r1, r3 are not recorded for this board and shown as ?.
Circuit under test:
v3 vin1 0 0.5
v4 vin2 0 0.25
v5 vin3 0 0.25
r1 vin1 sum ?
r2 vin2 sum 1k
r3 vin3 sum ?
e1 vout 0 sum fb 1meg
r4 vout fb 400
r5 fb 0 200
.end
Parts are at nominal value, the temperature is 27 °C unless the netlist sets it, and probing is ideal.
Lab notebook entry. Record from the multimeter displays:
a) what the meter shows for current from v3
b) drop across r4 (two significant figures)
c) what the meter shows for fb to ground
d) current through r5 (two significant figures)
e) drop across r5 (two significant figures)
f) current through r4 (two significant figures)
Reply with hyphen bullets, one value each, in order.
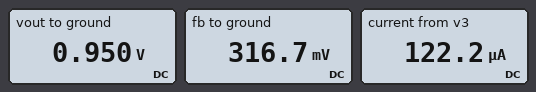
- 122.2 µA
- 630 mV
- 316.7 mV
- 1.6 mA
- 320 mV
- 1.6 mA
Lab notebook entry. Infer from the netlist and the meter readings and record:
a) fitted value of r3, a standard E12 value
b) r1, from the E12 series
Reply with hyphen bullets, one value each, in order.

- 1.2 kΩ
- 1.5 kΩ
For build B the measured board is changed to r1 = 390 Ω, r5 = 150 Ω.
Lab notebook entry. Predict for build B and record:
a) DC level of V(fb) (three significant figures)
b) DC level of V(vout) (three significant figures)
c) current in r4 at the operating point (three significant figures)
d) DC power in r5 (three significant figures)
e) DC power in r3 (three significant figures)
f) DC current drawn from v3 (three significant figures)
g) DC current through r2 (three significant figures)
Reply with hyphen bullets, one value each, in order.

- 396 mV
- 1.45 V
- 2.64 mA
- 1.04 mW
- 17.7 µW
- 267 µA
- 146 µA
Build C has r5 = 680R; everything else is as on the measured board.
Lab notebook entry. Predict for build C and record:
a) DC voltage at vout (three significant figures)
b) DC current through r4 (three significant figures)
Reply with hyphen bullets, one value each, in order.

- 503 mV
- 466 µA
